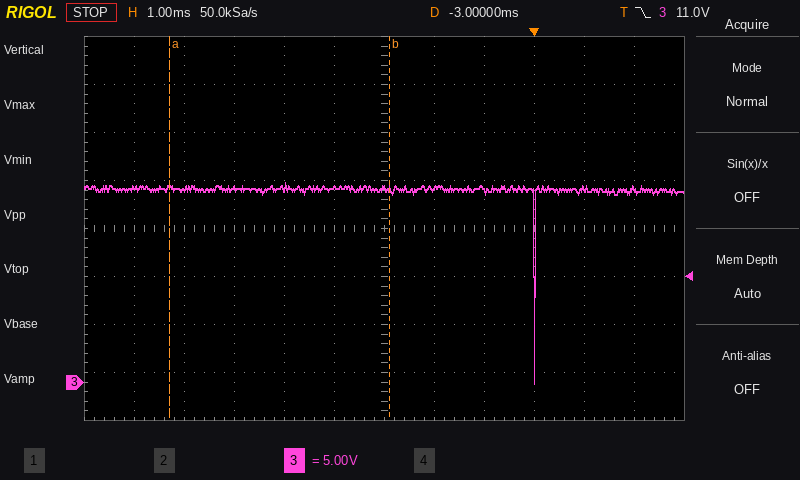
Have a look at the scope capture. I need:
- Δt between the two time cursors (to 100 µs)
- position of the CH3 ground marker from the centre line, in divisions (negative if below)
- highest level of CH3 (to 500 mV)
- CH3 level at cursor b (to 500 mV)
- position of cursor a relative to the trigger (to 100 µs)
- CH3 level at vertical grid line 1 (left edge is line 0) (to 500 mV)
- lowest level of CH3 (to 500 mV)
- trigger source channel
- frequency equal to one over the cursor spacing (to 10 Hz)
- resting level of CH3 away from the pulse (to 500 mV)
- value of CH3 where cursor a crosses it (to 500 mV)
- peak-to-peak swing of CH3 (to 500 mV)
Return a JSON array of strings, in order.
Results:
["4.4 ms", "-3.2 div", "21.0 V", "20.0 V", "-7.3 ms", "20.0 V", "0.0 V", "CH3", "230 Hz", "20.0 V", "20.0 V", "21.0 V"]
